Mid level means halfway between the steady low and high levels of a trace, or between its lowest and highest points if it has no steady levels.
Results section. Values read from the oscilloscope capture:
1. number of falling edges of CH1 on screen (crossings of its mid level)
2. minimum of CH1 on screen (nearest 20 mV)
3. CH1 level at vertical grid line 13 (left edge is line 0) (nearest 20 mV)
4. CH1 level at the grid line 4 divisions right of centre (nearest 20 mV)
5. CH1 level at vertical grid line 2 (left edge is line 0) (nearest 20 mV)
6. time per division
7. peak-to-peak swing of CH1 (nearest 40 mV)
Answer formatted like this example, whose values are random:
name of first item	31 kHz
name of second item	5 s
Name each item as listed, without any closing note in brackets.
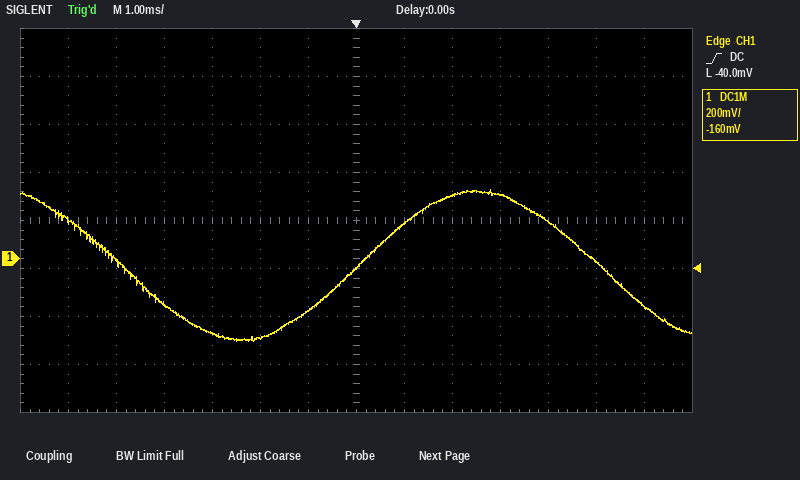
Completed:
number of falling edges of CH1 on screen	2
minimum of CH1 on screen	-340 mV
CH1 level at vertical grid line 13 (left edge is line 0)	-200 mV
CH1 level at the grid line 4 divisions right of centre	160 mV
CH1 level at vertical grid line 2 (left edge is line 0)	-20 mV
time per division	1 ms
peak-to-peak swing of CH1	640 mV
